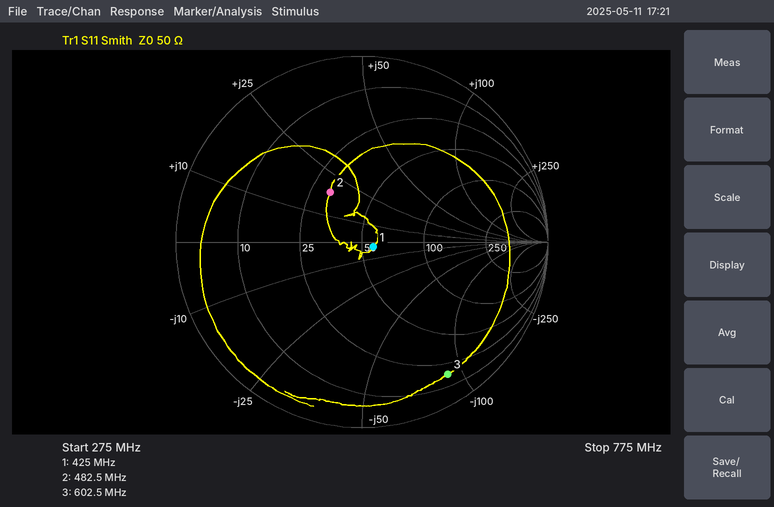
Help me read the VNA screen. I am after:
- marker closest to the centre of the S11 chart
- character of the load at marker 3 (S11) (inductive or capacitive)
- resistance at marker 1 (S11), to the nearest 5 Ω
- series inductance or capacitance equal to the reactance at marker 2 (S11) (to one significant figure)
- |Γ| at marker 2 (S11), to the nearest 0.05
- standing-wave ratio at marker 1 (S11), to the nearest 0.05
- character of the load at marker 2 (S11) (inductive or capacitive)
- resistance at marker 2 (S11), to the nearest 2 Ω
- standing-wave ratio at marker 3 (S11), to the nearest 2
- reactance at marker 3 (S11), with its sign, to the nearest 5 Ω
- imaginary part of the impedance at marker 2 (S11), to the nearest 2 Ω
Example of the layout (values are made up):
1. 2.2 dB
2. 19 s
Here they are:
1. marker 1
2. capacitive
3. 55 Ω
4. 6 nH
5. 0.30
6. 1.15
7. inductive
8. 32 Ω
9. 12
10. -90 Ω
11. +18 Ω
